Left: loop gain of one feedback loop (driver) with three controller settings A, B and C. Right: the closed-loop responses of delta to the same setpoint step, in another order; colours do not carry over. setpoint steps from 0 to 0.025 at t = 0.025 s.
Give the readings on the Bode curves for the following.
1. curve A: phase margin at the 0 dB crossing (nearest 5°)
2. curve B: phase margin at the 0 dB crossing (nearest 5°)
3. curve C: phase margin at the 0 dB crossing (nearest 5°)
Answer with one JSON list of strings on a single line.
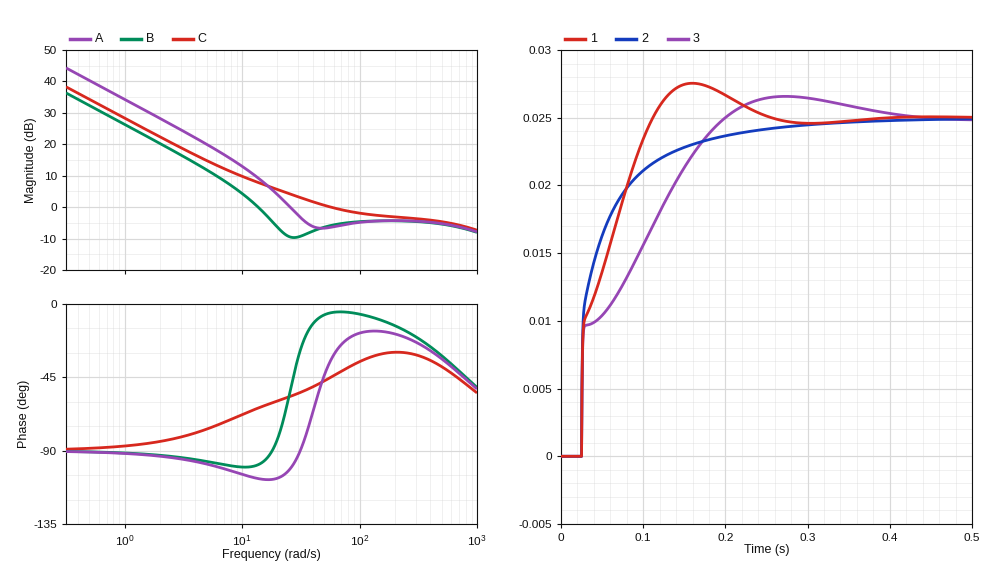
["80°", "80°", "135°"]
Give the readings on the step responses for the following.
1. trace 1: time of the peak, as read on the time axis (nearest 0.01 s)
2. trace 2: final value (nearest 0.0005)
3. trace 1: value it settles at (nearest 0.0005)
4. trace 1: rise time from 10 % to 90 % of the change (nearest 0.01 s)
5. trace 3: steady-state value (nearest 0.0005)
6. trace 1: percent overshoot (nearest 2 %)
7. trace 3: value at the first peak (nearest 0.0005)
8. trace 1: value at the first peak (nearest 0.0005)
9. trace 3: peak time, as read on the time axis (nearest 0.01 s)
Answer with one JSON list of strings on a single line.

["0.16 s", "0.0250", "0.0250", "0.07 s", "0.0250", "10 %", "0.0265", "0.0275", "0.27 s"]
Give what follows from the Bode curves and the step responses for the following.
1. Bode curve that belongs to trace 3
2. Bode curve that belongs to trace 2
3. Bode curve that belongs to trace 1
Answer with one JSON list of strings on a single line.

["B", "C", "A"]
